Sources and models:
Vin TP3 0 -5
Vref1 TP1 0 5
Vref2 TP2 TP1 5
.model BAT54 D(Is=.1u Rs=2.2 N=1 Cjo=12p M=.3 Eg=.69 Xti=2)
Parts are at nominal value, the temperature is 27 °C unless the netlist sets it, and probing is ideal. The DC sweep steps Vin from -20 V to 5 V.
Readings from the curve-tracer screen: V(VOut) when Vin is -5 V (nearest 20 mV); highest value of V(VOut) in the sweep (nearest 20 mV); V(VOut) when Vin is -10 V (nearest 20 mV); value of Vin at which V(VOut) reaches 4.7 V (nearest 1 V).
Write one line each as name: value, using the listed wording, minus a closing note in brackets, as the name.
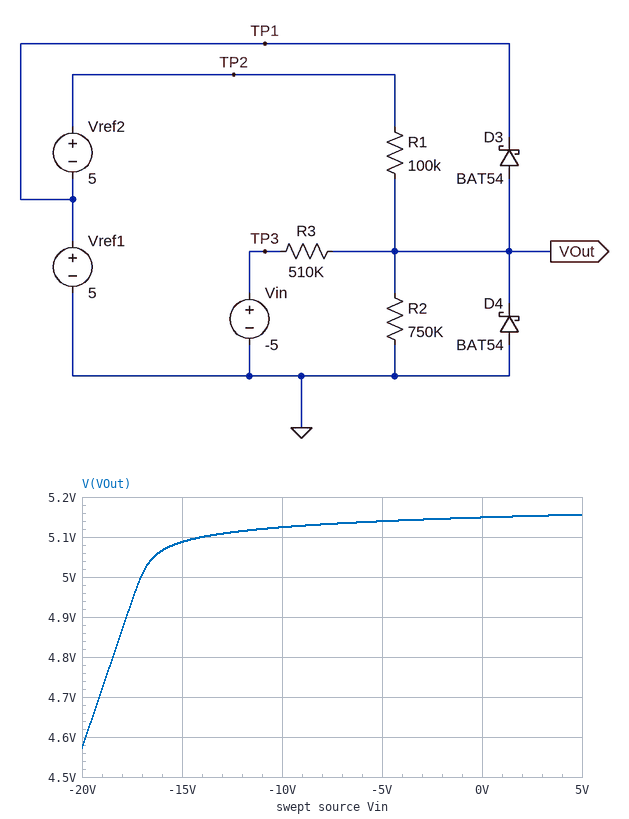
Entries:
V(VOut) when Vin is -5 V: 5.14 V
highest value of V(VOut) in the sweep: 5.16 V
V(VOut) when Vin is -10 V: 5.12 V
value of Vin at which V(VOut) reaches 4.7 V: -19 V
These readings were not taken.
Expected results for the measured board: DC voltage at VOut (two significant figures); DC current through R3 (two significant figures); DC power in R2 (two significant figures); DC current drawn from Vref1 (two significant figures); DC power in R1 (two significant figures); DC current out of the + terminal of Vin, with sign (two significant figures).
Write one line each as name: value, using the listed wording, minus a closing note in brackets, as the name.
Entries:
DC voltage at VOut: 5.1 V
DC current through R3: 20 µA
DC power in R2: 35 µW
DC current drawn from Vref1: 27 µA
DC power in R1: 240 µW
DC current out of the + terminal of Vin, with sign: -20 µA
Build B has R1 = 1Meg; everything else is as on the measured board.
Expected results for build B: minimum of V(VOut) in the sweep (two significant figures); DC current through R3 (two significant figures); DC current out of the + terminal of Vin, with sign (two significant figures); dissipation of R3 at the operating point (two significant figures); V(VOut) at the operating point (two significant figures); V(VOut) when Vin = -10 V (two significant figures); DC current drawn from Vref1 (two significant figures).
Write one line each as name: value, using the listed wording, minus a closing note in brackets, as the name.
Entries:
minimum of V(VOut) in the sweep: -150 mV
DC current through R3: 9.9 µA
DC current out of the + terminal of Vin, with sign: -9.9 µA
dissipation of R3 at the operating point: 50 µW
V(VOut) at the operating point: 49 mV
V(VOut) when Vin = -10 V: -120 mV
DC current drawn from Vref1: 10 µA
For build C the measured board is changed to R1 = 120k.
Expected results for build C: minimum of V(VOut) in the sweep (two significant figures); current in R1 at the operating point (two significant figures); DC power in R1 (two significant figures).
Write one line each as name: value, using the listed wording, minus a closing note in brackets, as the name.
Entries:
minimum of V(VOut) in the sweep: 3.8 V
current in R1 at the operating point: 41 µA
DC power in R1: 200 µW
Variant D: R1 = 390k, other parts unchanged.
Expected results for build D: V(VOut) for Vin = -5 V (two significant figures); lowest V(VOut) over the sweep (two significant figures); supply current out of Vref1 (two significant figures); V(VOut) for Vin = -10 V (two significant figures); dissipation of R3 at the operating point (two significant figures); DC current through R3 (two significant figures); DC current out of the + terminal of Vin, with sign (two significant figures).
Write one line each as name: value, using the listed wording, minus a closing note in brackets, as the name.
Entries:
V(VOut) for Vin = -5 V: 2.7 V
lowest V(VOut) over the sweep: -130 mV
supply current out of Vref1: 19 µA
V(VOut) for Vin = -10 V: 1.0 V
dissipation of R3 at the operating point: 120 µW
DC current through R3: 15 µA
DC current out of the + terminal of Vin, with sign: -15 µA
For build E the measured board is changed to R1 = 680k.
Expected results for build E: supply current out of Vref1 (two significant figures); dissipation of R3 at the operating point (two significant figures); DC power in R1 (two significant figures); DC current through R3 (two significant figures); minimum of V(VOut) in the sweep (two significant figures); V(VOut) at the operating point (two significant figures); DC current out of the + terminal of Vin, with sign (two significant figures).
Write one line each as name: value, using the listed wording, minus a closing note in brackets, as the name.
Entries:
supply current out of Vref1: 13 µA
dissipation of R3 at the operating point: 71 µW
DC power in R1: 120 µW
DC current through R3: 12 µA
minimum of V(VOut) in the sweep: -140 mV
V(VOut) at the operating point: 1.0 V
DC current out of the + terminal of Vin, with sign: -12 µA
